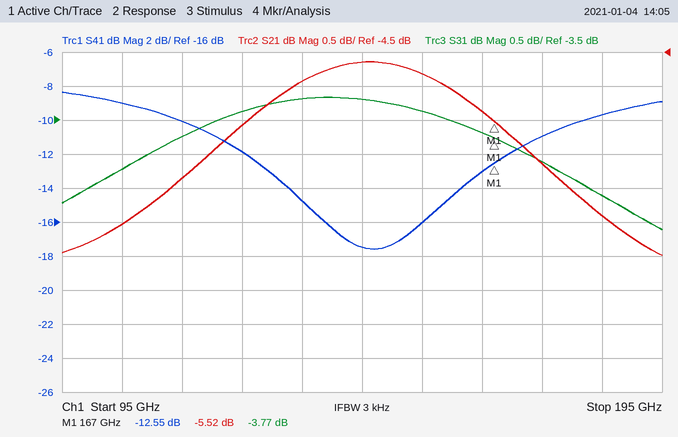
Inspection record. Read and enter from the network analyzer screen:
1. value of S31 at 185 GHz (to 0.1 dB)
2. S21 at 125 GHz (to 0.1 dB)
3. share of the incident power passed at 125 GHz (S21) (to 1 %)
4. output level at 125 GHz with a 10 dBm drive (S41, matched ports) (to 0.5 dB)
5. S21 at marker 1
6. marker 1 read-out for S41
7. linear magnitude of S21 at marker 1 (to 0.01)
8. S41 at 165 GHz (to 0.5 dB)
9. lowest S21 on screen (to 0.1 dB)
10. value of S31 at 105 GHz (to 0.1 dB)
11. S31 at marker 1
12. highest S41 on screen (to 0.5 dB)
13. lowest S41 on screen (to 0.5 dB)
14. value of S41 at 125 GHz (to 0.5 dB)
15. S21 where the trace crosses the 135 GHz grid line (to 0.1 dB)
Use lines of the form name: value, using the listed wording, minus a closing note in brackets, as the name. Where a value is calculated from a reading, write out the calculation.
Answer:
value of S31 at 185 GHz: -4.6 dB
S21 at 125 GHz: -5.6 dB
share of the incident power passed at 125 GHz (S21): 10^(-5.6/10) ≈ 28 %
output level at 125 GHz with a 10 dBm drive (S41, matched ports): 10 dBm + (-12.0 dB) = -2.0 dBm
S21 at marker 1: -5.52 dB
marker 1 read-out for S41: -12.55 dB
linear magnitude of S21 at marker 1: 10^(-5.52/20) ≈ 0.53
S41 at 165 GHz: -13.0 dB
lowest S21 on screen: -7.5 dB
value of S31 at 105 GHz: -4.2 dB
S31 at marker 1: -3.77 dB
highest S41 on screen: -8.5 dB
lowest S41 on screen: -17.5 dB
value of S41 at 125 GHz: -12.0 dB
S21 where the trace crosses the 135 GHz grid line: -4.9 dB
